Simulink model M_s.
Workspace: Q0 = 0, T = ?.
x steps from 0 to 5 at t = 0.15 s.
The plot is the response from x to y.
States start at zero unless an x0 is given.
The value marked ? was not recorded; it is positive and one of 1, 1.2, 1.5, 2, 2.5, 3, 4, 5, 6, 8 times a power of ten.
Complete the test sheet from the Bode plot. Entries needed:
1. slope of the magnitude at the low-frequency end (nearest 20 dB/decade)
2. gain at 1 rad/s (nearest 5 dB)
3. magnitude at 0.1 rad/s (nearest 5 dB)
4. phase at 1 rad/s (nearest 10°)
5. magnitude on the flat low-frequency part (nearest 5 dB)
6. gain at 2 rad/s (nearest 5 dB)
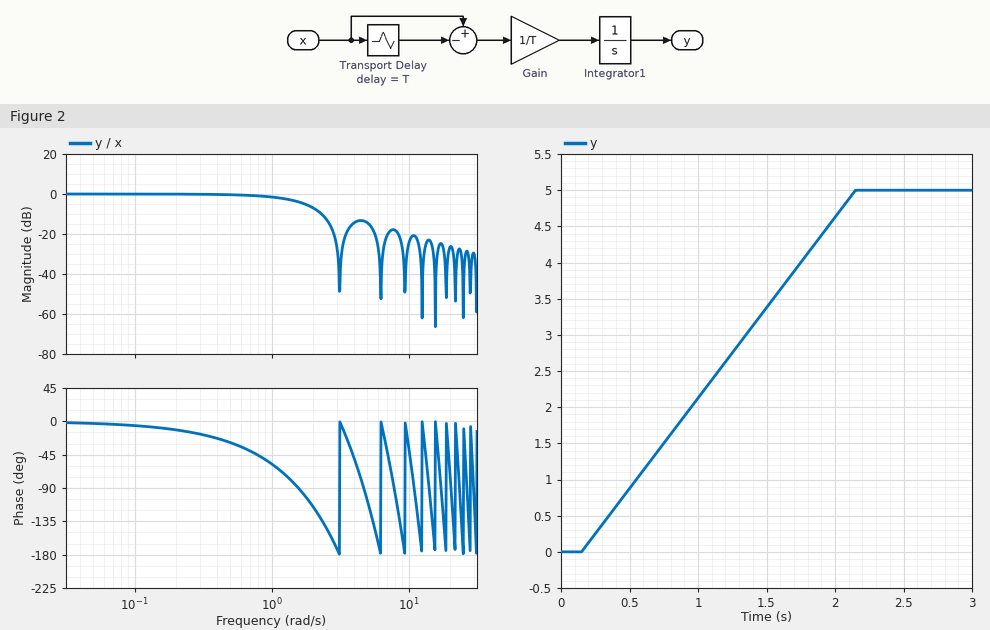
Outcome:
0 dB/decade
0 dB
0 dB
-60°
0 dB
-5 dB
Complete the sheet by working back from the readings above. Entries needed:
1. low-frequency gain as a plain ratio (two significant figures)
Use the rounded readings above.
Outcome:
1.0
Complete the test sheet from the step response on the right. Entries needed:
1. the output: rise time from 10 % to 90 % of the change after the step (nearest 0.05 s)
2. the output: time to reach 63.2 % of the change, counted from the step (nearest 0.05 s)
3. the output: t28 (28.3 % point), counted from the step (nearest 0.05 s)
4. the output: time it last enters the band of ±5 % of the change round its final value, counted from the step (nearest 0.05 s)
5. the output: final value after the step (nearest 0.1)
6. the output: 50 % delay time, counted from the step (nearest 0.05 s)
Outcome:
1.60 s
1.25 s
0.55 s
1.90 s
5.0
1.00 s
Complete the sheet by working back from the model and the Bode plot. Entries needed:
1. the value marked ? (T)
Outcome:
2
